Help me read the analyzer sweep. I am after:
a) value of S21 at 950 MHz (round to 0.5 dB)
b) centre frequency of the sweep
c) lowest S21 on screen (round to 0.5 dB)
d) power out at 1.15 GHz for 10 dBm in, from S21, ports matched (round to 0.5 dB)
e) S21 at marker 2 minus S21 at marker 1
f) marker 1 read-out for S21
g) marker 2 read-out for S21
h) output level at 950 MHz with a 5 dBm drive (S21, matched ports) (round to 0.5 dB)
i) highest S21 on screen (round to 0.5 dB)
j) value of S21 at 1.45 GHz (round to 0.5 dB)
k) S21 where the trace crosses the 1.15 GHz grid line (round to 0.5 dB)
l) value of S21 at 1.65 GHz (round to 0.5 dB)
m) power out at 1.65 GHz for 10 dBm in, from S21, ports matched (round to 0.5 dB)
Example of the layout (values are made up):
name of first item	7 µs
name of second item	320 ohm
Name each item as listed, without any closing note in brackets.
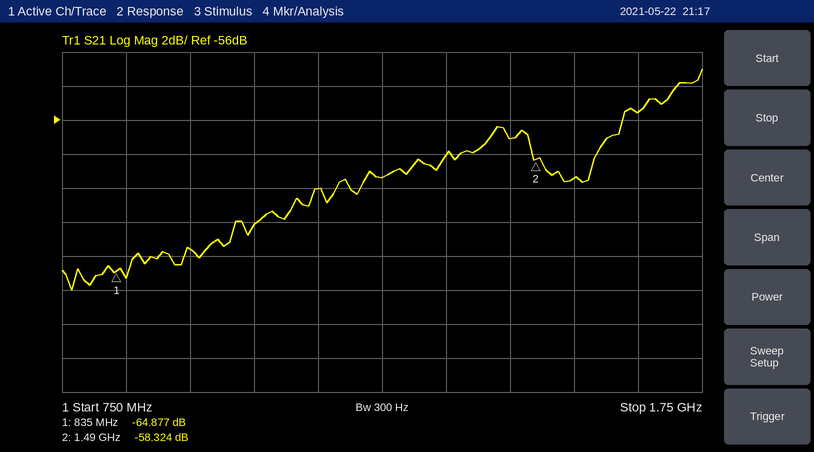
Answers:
value of S21 at 950 MHz	-63.5 dB
centre frequency of the sweep	1.25 GHz
lowest S21 on screen	-66.0 dB
power out at 1.15 GHz for 10 dBm in, from S21, ports matched	-50.0 dBm
S21 at marker 2 minus S21 at marker 1	6.553 dB
marker 1 read-out for S21	-64.877 dB
marker 2 read-out for S21	-58.324 dB
output level at 950 MHz with a 5 dBm drive (S21, matched ports)	-58.5 dBm
highest S21 on screen	-53.0 dB
value of S21 at 1.45 GHz	-57.0 dB
S21 where the trace crosses the 1.15 GHz grid line	-60.0 dB
value of S21 at 1.65 GHz	-55.5 dB
power out at 1.65 GHz for 10 dBm in, from S21, ports matched	-45.5 dBm
